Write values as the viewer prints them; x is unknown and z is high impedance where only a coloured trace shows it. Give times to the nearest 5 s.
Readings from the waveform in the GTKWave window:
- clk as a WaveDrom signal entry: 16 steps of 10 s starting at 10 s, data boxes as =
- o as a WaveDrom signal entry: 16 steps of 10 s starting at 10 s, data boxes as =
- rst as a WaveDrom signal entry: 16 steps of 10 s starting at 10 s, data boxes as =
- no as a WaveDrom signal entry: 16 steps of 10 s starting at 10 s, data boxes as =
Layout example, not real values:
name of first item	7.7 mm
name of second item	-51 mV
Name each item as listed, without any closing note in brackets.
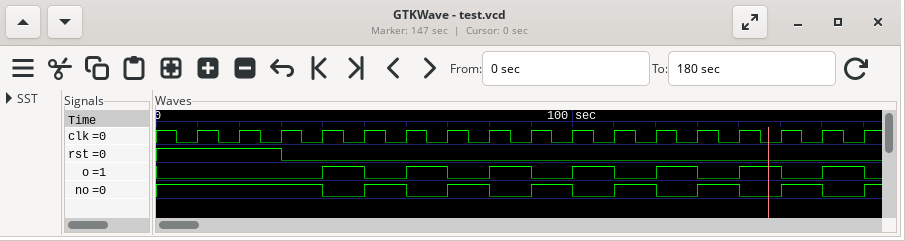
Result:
clk as a WaveDrom signal entry: 16 steps of 10 s starting at 10 s, data boxes as =	{name: 'clk', wave: 'p...............'}
o as a WaveDrom signal entry: 16 steps of 10 s starting at 10 s, data boxes as =	{name: 'o', wave: '0..1010101010101'}
rst as a WaveDrom signal entry: 16 steps of 10 s starting at 10 s, data boxes as =	{name: 'rst', wave: '1.0.............'}
no as a WaveDrom signal entry: 16 steps of 10 s starting at 10 s, data boxes as =	{name: 'no', wave: '1..0101010101010'}
